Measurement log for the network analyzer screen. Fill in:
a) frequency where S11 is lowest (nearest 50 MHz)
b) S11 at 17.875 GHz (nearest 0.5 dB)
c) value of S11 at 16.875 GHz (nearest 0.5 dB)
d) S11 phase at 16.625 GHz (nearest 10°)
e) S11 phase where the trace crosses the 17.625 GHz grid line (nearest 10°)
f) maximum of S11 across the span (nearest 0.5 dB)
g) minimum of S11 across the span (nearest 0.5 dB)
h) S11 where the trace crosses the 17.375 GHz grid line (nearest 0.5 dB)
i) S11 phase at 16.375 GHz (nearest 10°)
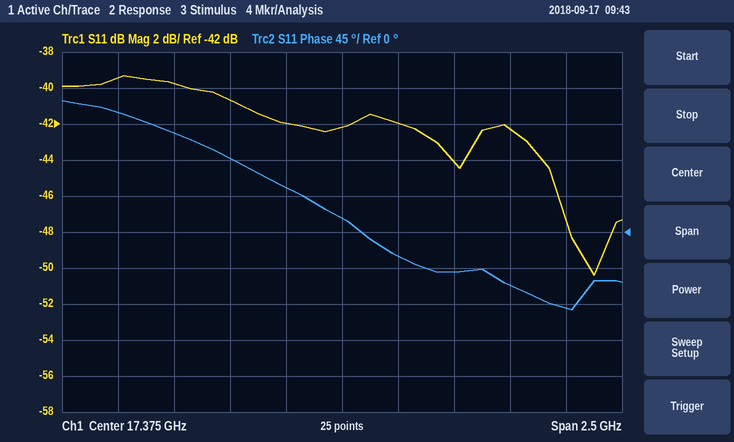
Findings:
18.50 GHz
-44.0 dB
-40.5 dB
120°
-30°
-39.5 dB
-50.5 dB
-42.0 dB
150°
